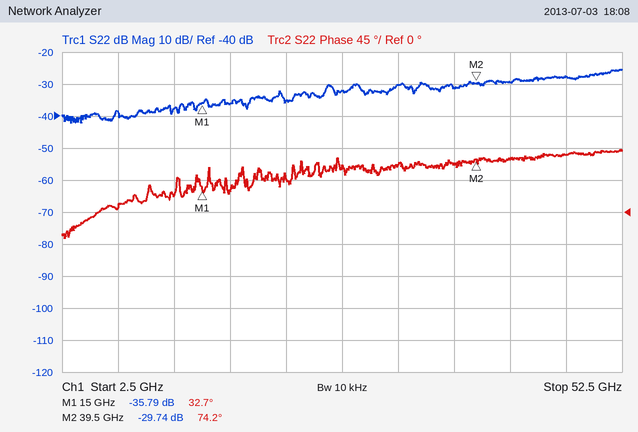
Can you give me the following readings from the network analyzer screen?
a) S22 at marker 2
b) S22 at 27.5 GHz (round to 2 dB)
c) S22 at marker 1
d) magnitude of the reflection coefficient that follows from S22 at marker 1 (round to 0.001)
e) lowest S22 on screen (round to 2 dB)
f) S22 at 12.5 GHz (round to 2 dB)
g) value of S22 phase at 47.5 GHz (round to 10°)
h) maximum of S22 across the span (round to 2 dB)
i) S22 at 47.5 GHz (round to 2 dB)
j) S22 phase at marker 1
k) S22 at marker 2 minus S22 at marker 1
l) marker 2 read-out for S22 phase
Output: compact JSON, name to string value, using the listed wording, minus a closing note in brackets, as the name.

{"S22 at marker 2": "-29.74 dB", "S22 at 27.5 GHz": "-32 dB", "S22 at marker 1": "-35.79 dB", "magnitude of the reflection coefficient that follows from S22 at marker 1": "0.016", "lowest S22 on screen": "-42 dB", "S22 at 12.5 GHz": "-38 dB", "value of S22 phase at 47.5 GHz": "80°", "maximum of S22 across the span": "-26 dB", "S22 at 47.5 GHz": "-28 dB", "S22 phase at marker 1": "32.7°", "S22 at marker 2 minus S22 at marker 1": "6.05 dB", "marker 2 read-out for S22 phase": "74.2°"}
